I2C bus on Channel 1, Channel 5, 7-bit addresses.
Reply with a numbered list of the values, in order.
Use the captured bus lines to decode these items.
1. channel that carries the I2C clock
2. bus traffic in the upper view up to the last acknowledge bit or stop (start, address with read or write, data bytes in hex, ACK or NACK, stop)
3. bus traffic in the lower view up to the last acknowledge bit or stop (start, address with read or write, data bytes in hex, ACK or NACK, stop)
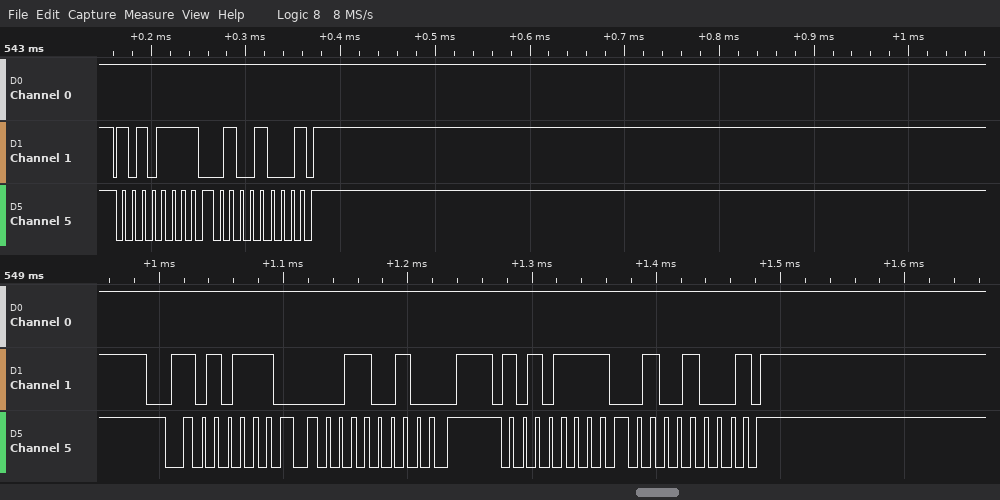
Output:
1. Channel 5
2. start, address 57 read ACK, 48 NACK, stop
3. start, address 57 write ACK, 32 ACK, stop, start, address 57 read ACK, 48 NACK, stop
